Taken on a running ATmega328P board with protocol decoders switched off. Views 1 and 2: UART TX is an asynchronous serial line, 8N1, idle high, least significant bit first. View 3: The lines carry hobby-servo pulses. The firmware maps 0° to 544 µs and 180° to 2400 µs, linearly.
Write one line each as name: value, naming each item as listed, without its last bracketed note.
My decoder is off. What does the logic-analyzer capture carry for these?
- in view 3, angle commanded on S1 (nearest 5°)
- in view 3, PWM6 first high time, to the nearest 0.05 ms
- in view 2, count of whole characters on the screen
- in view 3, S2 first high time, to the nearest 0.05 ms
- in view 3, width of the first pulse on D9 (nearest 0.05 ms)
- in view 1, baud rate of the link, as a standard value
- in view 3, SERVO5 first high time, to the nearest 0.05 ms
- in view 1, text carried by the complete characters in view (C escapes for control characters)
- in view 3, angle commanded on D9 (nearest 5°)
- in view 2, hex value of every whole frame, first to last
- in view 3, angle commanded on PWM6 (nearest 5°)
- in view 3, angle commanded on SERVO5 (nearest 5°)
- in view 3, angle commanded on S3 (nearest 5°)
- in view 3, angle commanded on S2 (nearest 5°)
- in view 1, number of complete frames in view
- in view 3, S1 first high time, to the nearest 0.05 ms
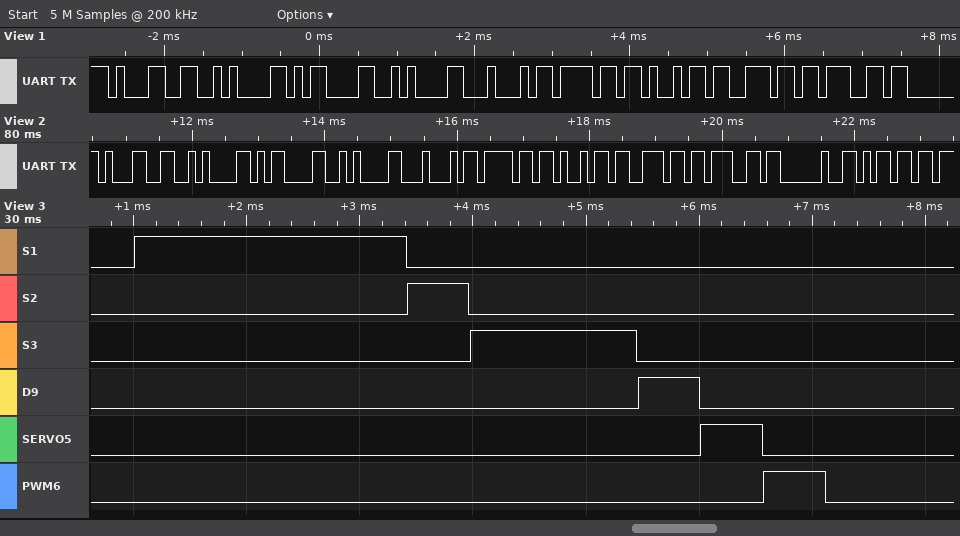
in view 3, angle commanded on S1: 180°
in view 3, PWM6 first high time, to the nearest 0.05 ms: 0.55 ms
in view 2, count of whole characters on the screen: 11
in view 3, S2 first high time, to the nearest 0.05 ms: 0.55 ms
in view 3, width of the first pulse on D9: 0.55 ms
in view 1, baud rate of the link, as a standard value: 9600 baud
in view 3, SERVO5 first high time, to the nearest 0.05 ms: 0.55 ms
in view 1, text carried by the complete characters in view: "1\n\r\nDoing"
in view 3, angle commanded on D9: 0°
in view 2, hex value of every whole frame, first to last: 31 0A 0D 0A 44 6F 69 6E 67 20 6D
in view 3, angle commanded on PWM6: 0°
in view 3, angle commanded on SERVO5: 0°
in view 3, angle commanded on S3: 90°
in view 3, angle commanded on S2: 0°
in view 1, number of complete frames in view: 9
in view 3, S1 first high time, to the nearest 0.05 ms: 2.40 ms
